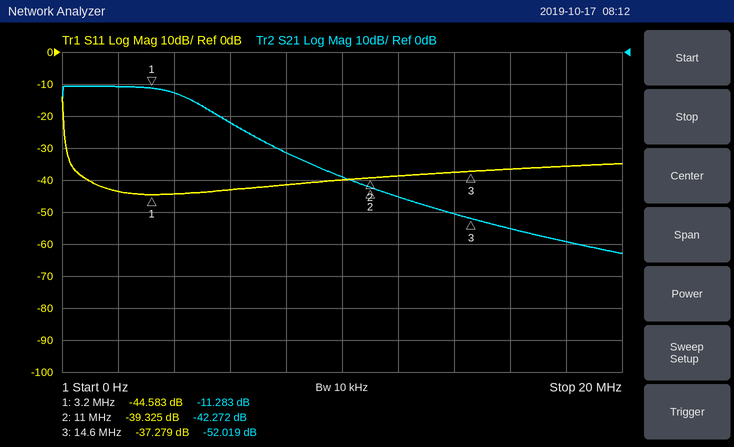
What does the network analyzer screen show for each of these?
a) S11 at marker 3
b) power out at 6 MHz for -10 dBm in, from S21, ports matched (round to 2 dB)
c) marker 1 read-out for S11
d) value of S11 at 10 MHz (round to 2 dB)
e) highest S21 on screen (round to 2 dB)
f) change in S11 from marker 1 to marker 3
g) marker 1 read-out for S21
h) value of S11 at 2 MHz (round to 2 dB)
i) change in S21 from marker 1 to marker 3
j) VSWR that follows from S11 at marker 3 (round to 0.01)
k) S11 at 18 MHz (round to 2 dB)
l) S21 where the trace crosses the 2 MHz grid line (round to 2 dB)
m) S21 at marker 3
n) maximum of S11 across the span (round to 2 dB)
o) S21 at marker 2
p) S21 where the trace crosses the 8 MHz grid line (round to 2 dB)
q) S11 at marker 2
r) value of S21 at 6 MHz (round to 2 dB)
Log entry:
-37.279 dB
-32 dBm
-44.583 dB
-40 dB
-10 dB
7.304 dB
-11.283 dB
-44 dB
-40.736 dB
1.03
-36 dB
-10 dB
-52.019 dB
-14 dB
-42.272 dB
-32 dB
-39.325 dB
-22 dB
